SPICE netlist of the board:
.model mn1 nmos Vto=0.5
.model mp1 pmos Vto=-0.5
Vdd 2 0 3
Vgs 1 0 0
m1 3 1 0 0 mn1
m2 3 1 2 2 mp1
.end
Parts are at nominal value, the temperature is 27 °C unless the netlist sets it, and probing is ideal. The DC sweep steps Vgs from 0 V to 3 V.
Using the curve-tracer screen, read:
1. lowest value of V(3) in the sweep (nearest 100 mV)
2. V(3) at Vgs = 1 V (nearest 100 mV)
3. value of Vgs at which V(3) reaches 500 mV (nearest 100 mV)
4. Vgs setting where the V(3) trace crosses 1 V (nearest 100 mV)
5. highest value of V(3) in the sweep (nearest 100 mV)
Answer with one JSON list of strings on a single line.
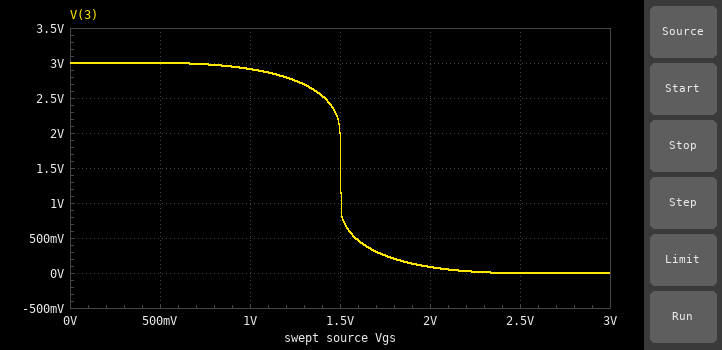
["0 V", "2.9 V", "1.6 V", "1.5 V", "3.0 V"]
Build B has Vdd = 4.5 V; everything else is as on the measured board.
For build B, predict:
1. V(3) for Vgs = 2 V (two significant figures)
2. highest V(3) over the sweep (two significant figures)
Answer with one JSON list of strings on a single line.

["3.8 V", "4.5 V"]
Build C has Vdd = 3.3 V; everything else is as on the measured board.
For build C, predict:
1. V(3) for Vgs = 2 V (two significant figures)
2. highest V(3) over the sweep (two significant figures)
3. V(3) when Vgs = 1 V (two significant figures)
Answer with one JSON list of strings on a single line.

["230 mV", "3.3 V", "3.2 V"]
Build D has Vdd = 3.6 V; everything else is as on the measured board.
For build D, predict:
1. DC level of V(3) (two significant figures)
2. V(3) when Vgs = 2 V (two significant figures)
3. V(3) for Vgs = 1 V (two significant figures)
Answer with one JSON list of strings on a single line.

["3.6 V", "480 mV", "3.5 V"]
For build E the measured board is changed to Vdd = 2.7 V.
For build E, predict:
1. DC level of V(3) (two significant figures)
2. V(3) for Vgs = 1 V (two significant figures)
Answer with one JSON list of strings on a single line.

["2.7 V", "2.6 V"]
